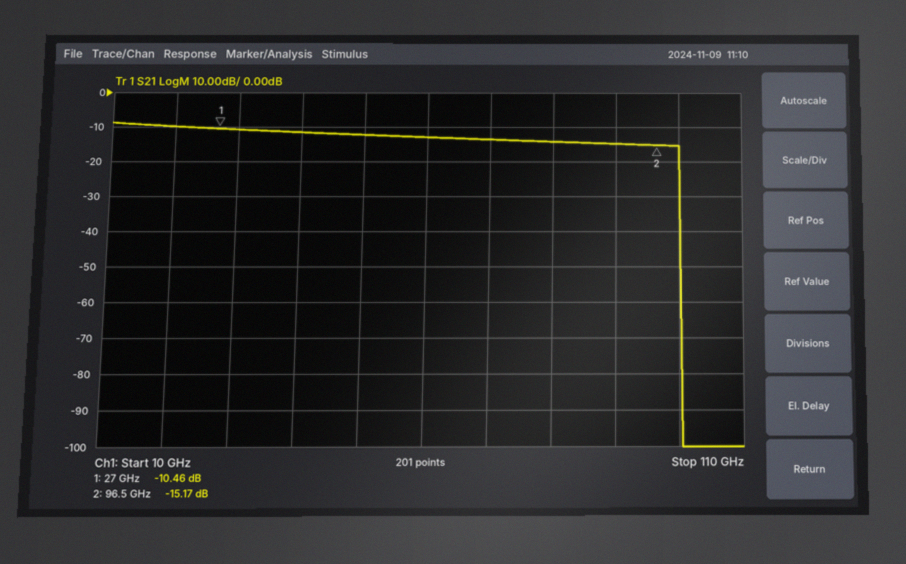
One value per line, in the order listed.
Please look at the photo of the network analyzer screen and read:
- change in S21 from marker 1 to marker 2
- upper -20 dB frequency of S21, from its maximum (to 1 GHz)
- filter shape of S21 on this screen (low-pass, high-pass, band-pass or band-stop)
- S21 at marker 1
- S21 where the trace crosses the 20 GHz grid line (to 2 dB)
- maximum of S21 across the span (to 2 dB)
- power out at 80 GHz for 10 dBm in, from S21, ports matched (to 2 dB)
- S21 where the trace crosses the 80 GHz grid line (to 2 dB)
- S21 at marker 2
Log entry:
-4.71 dB
100 GHz
low-pass
-10.46 dB
-10 dB
-8 dB
-4 dBm
-14 dB
-15.17 dB
